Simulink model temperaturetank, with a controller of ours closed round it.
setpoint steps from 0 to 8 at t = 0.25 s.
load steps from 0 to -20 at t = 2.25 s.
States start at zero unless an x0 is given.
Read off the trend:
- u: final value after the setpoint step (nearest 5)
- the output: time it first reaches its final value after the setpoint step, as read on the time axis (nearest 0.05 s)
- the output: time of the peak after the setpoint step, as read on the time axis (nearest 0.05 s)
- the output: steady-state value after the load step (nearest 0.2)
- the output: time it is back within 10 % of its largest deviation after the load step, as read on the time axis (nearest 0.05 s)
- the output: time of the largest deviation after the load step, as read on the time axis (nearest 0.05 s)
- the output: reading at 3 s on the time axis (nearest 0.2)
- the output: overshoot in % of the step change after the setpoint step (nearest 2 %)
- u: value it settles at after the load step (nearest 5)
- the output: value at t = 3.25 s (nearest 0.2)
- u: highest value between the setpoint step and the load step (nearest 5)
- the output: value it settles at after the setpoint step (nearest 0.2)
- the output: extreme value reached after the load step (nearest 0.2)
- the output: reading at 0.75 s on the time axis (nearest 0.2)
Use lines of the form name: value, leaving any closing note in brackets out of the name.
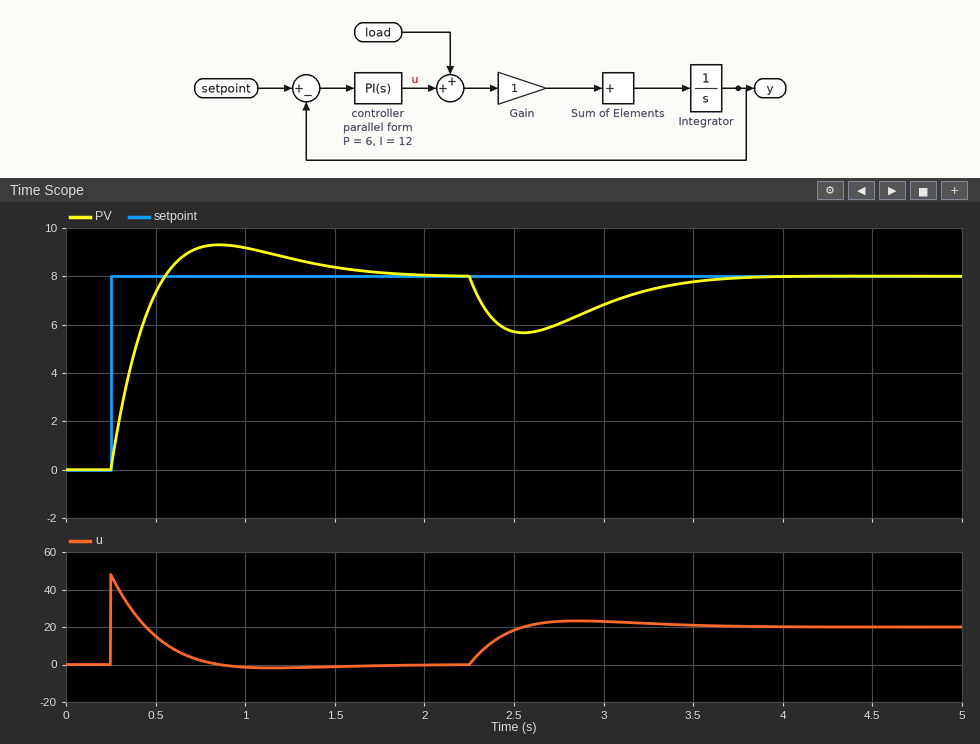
u: final value after the setpoint step: 0
the output: time it first reaches its final value after the setpoint step, as read on the time axis: 0.55 s
the output: time of the peak after the setpoint step, as read on the time axis: 0.85 s
the output: steady-state value after the load step: 8.0
the output: time it is back within 10 % of its largest deviation after the load step, as read on the time axis: 3.50 s
the output: time of the largest deviation after the load step, as read on the time axis: 2.55 s
the output: reading at 3 s on the time axis: 6.8
the output: overshoot in % of the step change after the setpoint step: 16 %
u: value it settles at after the load step: 20
the output: value at t = 3.25 s: 7.4
u: highest value between the setpoint step and the load step: 50
the output: value it settles at after the setpoint step: 8.0
the output: extreme value reached after the load step: 5.6
the output: reading at 0.75 s on the time axis: 9.2
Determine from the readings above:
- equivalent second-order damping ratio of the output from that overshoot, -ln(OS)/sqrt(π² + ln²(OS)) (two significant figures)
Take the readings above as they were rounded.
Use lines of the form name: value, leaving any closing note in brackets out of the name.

equivalent second-order damping ratio of the output from that overshoot, -ln(OS)/sqrt(π² + ln²(OS)): 0.50
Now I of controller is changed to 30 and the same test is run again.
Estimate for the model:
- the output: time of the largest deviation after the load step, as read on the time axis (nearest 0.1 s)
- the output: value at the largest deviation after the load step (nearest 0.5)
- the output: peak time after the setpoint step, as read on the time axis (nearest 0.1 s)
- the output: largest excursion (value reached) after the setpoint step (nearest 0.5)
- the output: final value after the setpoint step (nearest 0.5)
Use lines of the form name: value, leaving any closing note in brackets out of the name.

the output: time of the largest deviation after the load step, as read on the time axis: 2.5 s
the output: value at the largest deviation after the load step: 6.0
the output: peak time after the setpoint step, as read on the time axis: 0.7 s
the output: largest excursion (value reached) after the setpoint step: 10.0
the output: final value after the setpoint step: 8.0
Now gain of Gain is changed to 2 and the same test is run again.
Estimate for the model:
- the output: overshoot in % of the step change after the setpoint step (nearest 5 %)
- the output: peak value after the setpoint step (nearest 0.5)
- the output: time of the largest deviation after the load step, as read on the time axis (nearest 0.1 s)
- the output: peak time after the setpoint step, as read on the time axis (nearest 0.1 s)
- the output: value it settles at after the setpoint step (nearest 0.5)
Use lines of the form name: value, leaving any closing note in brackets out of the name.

the output: overshoot in % of the step change after the setpoint step: 10 %
the output: peak value after the setpoint step: 9.0
the output: time of the largest deviation after the load step, as read on the time axis: 2.4 s
the output: peak time after the setpoint step, as read on the time axis: 0.6 s
the output: value it settles at after the setpoint step: 8.0
